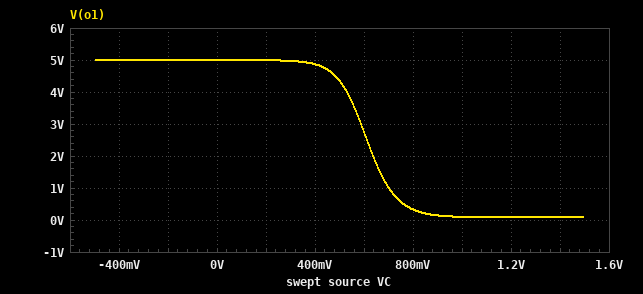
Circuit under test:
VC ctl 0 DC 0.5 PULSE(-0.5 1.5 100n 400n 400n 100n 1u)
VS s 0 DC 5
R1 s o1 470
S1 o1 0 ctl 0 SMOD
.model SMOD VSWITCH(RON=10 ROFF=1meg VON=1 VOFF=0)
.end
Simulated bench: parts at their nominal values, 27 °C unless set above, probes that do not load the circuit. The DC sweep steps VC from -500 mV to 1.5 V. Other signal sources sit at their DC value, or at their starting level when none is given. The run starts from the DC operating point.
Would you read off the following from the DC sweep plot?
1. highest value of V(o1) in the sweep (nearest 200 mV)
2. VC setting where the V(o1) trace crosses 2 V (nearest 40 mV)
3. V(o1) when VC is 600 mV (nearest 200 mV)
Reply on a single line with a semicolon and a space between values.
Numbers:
5.0 V; 640 mV; 2.8 V
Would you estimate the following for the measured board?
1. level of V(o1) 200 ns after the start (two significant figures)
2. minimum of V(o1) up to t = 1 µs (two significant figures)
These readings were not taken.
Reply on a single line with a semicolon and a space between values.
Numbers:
5.0 V; 100 mV
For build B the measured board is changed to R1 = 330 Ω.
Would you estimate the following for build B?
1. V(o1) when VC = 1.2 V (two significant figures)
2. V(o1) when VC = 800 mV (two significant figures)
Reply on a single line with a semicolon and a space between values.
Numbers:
150 mV; 460 mV
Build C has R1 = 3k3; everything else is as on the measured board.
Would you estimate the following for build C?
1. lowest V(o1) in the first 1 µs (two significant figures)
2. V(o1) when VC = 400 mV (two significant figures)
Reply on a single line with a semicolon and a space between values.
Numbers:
15 mV; 4.2 V
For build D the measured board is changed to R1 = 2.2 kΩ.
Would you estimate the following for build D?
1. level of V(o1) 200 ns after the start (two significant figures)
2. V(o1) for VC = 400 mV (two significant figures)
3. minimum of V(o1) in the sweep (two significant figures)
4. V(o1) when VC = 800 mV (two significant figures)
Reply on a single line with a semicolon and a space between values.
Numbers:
5.0 V; 4.4 V; 23 mV; 74 mV
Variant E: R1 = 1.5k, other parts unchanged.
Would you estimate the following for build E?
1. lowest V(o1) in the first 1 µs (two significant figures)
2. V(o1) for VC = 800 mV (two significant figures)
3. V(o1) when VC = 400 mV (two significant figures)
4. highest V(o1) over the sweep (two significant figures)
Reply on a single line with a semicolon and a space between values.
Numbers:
33 mV; 110 mV; 4.6 V; 5.0 V
